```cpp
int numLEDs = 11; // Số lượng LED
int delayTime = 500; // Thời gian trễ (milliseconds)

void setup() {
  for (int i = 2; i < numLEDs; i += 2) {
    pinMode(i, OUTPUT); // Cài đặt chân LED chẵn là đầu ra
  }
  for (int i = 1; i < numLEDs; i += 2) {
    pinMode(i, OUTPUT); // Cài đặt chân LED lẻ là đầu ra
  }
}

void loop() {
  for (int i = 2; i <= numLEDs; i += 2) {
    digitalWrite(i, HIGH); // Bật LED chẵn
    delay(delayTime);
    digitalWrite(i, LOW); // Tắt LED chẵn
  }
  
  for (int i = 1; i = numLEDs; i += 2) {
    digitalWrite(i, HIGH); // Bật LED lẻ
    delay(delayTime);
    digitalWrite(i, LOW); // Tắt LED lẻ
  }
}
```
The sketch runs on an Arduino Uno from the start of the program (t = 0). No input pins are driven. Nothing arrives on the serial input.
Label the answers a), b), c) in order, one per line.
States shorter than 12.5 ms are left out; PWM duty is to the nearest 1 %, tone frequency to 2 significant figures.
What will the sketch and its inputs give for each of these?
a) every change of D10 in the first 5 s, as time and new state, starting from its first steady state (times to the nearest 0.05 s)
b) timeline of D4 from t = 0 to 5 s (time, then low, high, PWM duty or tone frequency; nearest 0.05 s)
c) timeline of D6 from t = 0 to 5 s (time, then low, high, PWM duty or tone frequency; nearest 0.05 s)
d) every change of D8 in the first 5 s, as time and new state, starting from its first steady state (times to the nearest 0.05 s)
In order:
a) 0 s low; 2 s high; 2.5 s low
b) 0 s low; 0.5 s high; 1 s low
c) 0 s low; 1 s high; 1.5 s low
d) 0 s low; 1.5 s high; 2 s low
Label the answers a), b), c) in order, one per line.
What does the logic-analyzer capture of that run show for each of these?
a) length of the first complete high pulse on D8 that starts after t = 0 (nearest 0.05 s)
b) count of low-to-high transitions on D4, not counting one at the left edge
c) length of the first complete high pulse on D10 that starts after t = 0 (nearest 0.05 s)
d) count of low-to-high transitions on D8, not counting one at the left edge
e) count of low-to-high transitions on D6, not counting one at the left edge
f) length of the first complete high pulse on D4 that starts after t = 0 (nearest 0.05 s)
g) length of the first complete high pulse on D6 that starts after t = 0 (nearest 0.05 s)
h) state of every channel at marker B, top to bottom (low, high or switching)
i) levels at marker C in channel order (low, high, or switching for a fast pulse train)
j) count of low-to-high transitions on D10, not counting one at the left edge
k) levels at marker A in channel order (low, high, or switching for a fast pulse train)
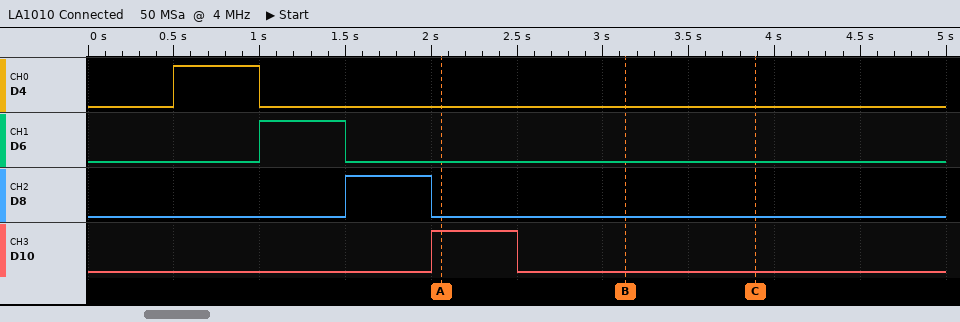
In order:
a) 0.50 s
b) 1
c) 0.50 s
d) 1
e) 1
f) 0.50 s
g) 0.50 s
h) D4 low, D6 low, D8 low, D10 low
i) D4 low, D6 low, D8 low, D10 low
j) 1
k) D4 low, D6 low, D8 low, D10 high
